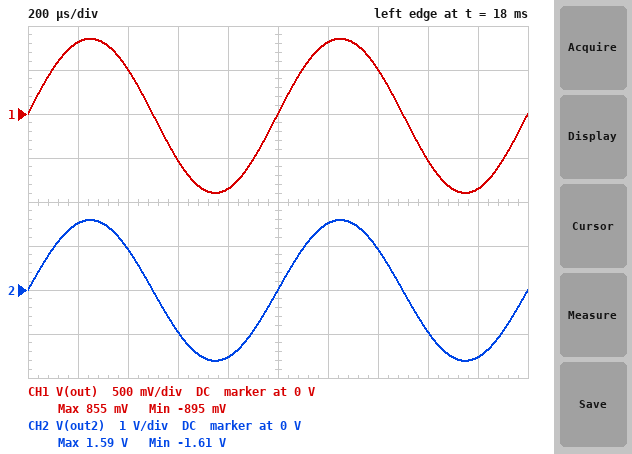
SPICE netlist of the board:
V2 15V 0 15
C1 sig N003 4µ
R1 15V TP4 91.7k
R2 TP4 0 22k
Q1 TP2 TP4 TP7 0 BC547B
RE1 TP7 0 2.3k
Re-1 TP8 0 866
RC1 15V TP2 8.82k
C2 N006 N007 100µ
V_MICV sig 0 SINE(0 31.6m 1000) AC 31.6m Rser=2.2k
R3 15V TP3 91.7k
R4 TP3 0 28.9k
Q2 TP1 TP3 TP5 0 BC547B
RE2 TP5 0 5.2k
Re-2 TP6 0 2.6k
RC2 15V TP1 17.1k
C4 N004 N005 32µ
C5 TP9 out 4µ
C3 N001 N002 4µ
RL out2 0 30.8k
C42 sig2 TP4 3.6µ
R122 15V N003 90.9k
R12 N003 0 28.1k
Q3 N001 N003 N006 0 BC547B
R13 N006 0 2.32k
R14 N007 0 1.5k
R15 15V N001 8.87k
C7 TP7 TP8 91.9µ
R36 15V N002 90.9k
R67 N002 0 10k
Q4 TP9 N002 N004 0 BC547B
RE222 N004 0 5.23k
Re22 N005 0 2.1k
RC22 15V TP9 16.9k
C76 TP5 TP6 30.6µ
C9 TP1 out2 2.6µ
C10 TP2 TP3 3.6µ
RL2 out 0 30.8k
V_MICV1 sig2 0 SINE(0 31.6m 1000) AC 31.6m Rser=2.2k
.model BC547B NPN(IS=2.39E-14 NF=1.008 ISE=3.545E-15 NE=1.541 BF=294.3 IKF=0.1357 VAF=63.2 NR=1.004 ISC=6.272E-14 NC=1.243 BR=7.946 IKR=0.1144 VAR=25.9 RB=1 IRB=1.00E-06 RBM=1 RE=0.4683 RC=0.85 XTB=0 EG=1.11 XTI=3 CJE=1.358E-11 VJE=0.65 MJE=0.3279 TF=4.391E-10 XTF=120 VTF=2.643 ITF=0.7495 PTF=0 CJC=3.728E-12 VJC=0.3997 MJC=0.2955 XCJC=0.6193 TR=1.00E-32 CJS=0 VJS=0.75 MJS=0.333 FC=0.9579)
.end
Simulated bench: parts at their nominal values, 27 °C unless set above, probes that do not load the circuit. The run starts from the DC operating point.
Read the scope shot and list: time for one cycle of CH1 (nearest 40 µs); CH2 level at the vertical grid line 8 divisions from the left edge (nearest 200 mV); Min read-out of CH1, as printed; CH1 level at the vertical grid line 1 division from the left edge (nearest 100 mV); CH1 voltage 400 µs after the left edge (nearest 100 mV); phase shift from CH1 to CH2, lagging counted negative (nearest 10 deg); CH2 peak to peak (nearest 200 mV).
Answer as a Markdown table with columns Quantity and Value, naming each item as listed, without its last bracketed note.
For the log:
| Quantity | Value |
|---|---|
| time for one cycle of CH1 | 1.00 ms |
| CH2 level at the vertical grid line 8 divisions from the left edge | -1.0 V |
| Min read-out of CH1, as printed | -895 mV |
| CH1 level at the vertical grid line 1 division from the left edge | 800 mV |
| CH1 voltage 400 µs after the left edge | 500 mV |
| phase shift from CH1 to CH2, lagging counted negative | 0 deg |
| CH2 peak to peak | 3.2 V |
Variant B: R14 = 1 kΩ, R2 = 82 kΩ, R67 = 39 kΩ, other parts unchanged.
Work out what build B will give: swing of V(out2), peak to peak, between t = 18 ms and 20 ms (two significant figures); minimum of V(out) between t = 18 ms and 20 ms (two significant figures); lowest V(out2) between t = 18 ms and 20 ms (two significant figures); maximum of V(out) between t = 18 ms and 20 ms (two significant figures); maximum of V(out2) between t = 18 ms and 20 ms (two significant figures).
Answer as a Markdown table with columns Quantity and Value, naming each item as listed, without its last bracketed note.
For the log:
| Quantity | Value |
|---|---|
| swing of V(out2), peak to peak, between t = 18 ms and 20 ms | 41 mV |
| minimum of V(out) between t = 18 ms and 20 ms | -62 mV |
| lowest V(out2) between t = 18 ms and 20 ms | -22 mV |
| maximum of V(out) between t = 18 ms and 20 ms | 1.3 V |
| maximum of V(out2) between t = 18 ms and 20 ms | 19 mV |
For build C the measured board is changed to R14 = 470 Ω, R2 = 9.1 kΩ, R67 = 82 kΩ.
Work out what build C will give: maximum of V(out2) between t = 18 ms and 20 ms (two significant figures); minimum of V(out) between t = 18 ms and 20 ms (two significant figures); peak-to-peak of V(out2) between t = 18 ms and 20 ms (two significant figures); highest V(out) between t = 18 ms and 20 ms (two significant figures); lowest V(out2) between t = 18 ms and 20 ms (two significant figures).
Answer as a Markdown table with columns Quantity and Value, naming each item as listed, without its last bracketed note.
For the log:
| Quantity | Value |
|---|---|
| maximum of V(out2) between t = 18 ms and 20 ms | 1.3 V |
| minimum of V(out) between t = 18 ms and 20 ms | -36 mV |
| peak-to-peak of V(out2) between t = 18 ms and 20 ms | 2.6 V |
| highest V(out) between t = 18 ms and 20 ms | 65 mV |
| lowest V(out2) between t = 18 ms and 20 ms | -1.3 V |
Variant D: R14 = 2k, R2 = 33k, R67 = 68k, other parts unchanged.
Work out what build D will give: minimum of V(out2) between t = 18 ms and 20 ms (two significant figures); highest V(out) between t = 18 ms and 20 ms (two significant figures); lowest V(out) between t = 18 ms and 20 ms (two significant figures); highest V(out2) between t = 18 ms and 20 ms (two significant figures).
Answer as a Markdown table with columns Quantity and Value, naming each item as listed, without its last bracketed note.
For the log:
| Quantity | Value |
|---|---|
| minimum of V(out2) between t = 18 ms and 20 ms | -1.0 V |
| highest V(out) between t = 18 ms and 20 ms | 23 mV |
| lowest V(out) between t = 18 ms and 20 ms | -19 mV |
| highest V(out2) between t = 18 ms and 20 ms | 240 mV |
